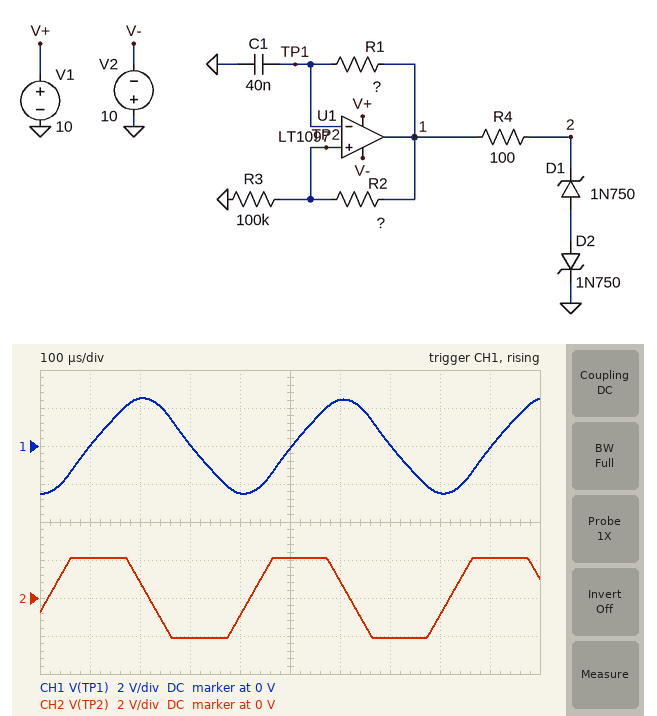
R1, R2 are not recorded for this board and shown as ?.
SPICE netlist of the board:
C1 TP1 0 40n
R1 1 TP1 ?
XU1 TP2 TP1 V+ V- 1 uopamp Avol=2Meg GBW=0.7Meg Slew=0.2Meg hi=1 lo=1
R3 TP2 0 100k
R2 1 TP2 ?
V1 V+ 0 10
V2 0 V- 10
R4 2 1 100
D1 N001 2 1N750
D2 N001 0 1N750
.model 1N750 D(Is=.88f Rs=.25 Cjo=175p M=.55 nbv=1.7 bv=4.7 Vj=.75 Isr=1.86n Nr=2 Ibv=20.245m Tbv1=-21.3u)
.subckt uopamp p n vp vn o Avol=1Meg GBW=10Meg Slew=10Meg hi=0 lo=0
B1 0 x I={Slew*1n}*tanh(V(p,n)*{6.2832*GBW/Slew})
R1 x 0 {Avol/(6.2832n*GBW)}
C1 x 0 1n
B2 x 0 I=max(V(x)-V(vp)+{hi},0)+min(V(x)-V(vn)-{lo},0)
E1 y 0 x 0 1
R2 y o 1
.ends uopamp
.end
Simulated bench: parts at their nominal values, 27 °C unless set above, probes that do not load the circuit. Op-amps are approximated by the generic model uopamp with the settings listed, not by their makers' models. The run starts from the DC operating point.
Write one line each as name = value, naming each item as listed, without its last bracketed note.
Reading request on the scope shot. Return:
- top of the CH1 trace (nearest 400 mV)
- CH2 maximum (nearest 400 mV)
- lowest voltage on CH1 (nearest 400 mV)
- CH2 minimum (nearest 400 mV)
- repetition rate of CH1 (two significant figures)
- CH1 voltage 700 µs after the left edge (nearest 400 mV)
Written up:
top of the CH1 trace = 2.4 V
CH2 maximum = 2.0 V
lowest voltage on CH1 = -2.4 V
CH2 minimum = -2.0 V
repetition rate of CH1 = 2.5 kHz
CH1 voltage 700 µs after the left edge = 0 V
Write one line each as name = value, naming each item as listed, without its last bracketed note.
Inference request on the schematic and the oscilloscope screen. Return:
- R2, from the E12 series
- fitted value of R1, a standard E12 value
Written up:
R2, from the E12 series = 330 kΩ
fitted value of R1, a standard E12 value = 6.8 kΩ
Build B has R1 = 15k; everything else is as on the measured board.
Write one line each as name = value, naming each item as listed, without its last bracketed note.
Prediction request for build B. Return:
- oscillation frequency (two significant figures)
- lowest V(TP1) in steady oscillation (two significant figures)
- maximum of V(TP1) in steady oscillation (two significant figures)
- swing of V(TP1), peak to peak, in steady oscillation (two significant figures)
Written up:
oscillation frequency = 1.4 kHz
lowest V(TP1) in steady oscillation = -2.3 V
maximum of V(TP1) in steady oscillation = 2.3 V
swing of V(TP1), peak to peak, in steady oscillation = 4.6 V
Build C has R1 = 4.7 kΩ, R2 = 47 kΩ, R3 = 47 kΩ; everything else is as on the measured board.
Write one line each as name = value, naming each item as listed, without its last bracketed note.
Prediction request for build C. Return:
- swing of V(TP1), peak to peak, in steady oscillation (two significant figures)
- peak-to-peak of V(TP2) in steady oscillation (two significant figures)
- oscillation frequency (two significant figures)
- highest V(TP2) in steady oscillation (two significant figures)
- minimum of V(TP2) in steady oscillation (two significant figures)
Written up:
swing of V(TP1), peak to peak, in steady oscillation = 9.5 V
peak-to-peak of V(TP2) in steady oscillation = 9.0 V
oscillation frequency = 1.9 kHz
highest V(TP2) in steady oscillation = 4.5 V
minimum of V(TP2) in steady oscillation = -4.5 V
